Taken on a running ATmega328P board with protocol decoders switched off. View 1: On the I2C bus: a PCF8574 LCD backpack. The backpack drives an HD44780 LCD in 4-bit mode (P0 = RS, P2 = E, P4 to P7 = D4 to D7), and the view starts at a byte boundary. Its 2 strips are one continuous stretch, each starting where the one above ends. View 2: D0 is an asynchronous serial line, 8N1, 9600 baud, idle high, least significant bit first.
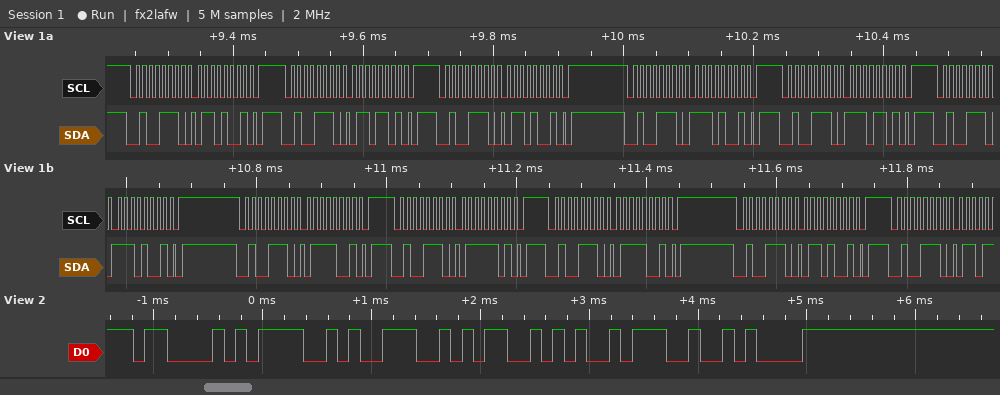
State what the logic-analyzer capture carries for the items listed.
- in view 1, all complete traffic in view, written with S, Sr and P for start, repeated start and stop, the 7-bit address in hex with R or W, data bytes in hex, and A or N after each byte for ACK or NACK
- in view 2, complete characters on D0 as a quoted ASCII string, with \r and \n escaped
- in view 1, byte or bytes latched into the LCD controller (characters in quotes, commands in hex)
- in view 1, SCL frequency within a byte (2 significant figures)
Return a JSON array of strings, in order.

["S 27W A 69 A P S 27W A 6D A P S 27W A 69 A P S 27W A E9 A P S 27W A ED A P S 27W A E9 A P S 27W A 79 A P S 27W A 7D A P S 27W A 79 A P S 27W A 69 A P S 27W A", "\"CONS:\\n\"", "'n'", "100 kHz"]
